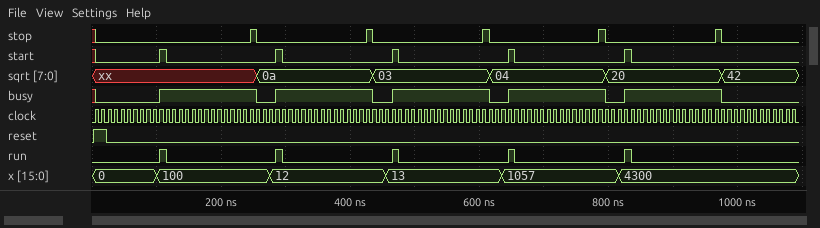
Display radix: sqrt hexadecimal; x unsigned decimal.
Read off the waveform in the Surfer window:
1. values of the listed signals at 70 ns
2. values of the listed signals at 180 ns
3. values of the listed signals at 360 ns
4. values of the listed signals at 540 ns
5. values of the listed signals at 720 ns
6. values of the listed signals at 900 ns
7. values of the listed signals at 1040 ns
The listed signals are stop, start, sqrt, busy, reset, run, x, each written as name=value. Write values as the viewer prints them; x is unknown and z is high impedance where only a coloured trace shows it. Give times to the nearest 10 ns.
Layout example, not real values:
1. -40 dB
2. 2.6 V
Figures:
1. stop=0, start=0, sqrt=xx, busy=0, reset=0, run=0, x=0
2. stop=0, start=0, sqrt=xx, busy=1, reset=0, run=0, x=100
3. stop=0, start=0, sqrt=0a, busy=1, reset=0, run=0, x=12
4. stop=0, start=0, sqrt=03, busy=1, reset=0, run=0, x=13
5. stop=0, start=0, sqrt=04, busy=1, reset=0, run=0, x=1057
6. stop=0, start=0, sqrt=20, busy=1, reset=0, run=0, x=4300
7. stop=0, start=0, sqrt=42, busy=0, reset=0, run=0, x=4300
